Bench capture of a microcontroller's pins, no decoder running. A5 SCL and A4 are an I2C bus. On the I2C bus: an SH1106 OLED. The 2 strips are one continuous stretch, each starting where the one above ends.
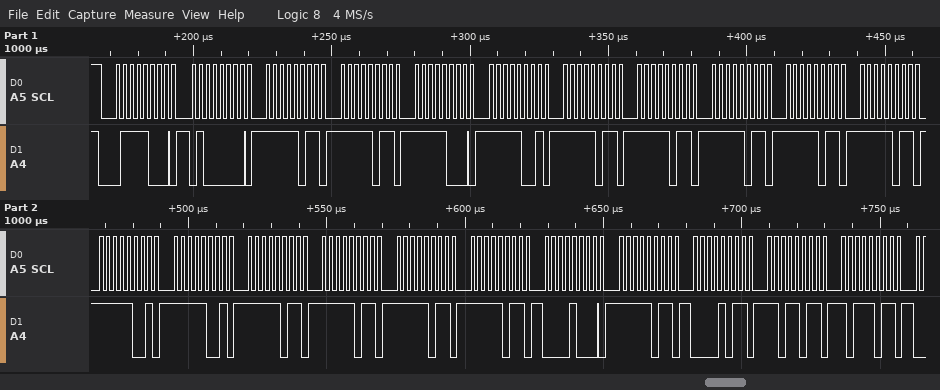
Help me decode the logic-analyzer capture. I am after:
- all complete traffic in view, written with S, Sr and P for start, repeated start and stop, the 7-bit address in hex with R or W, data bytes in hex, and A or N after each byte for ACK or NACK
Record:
S 3CW A 40 A FB A FB A F8 A F9 A FB A FB A FB A FB A FB A F9 A F9 A FB A FB A FB A FB A 08 A FB A 0B A DB A BB A
